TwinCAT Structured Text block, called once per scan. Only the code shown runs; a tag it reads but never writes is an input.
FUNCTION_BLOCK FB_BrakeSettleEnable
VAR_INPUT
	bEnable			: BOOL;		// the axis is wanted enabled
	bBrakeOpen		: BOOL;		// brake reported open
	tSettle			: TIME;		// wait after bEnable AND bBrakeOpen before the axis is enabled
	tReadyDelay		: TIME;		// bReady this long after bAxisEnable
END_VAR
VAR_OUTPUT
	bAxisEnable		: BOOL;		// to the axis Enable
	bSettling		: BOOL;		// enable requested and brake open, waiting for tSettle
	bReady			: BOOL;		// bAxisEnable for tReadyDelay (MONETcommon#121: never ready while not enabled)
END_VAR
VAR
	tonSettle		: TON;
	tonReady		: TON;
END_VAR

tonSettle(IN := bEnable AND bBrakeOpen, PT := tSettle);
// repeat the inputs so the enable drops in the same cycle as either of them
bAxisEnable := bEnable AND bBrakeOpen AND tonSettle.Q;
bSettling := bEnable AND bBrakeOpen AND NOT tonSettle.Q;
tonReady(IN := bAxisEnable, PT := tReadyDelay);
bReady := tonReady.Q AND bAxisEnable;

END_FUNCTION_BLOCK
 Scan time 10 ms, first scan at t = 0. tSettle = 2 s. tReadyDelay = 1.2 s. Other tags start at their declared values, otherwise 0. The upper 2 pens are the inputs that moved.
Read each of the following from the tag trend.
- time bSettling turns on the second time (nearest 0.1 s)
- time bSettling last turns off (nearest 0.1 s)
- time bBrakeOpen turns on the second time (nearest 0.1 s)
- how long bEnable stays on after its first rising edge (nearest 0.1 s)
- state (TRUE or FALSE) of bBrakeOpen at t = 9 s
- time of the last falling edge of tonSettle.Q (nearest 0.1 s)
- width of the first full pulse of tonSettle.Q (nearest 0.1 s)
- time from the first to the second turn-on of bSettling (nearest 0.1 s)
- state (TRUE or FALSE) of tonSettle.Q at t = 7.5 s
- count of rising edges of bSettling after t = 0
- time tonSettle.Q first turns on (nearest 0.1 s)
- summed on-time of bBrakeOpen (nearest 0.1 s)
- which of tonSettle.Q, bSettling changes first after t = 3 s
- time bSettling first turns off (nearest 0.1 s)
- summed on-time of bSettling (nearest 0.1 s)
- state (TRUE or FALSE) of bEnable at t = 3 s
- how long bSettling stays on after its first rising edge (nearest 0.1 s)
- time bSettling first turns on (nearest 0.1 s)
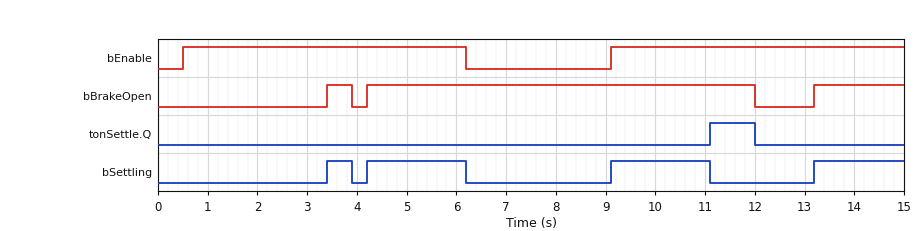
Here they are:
4.2 s
11.1 s
4.2 s
5.7 s
TRUE
12.0 s
0.9 s
0.8 s
FALSE
4
11.1 s
10.1 s
bSettling
3.9 s
6.3 s
TRUE
0.5 s
3.4 s
